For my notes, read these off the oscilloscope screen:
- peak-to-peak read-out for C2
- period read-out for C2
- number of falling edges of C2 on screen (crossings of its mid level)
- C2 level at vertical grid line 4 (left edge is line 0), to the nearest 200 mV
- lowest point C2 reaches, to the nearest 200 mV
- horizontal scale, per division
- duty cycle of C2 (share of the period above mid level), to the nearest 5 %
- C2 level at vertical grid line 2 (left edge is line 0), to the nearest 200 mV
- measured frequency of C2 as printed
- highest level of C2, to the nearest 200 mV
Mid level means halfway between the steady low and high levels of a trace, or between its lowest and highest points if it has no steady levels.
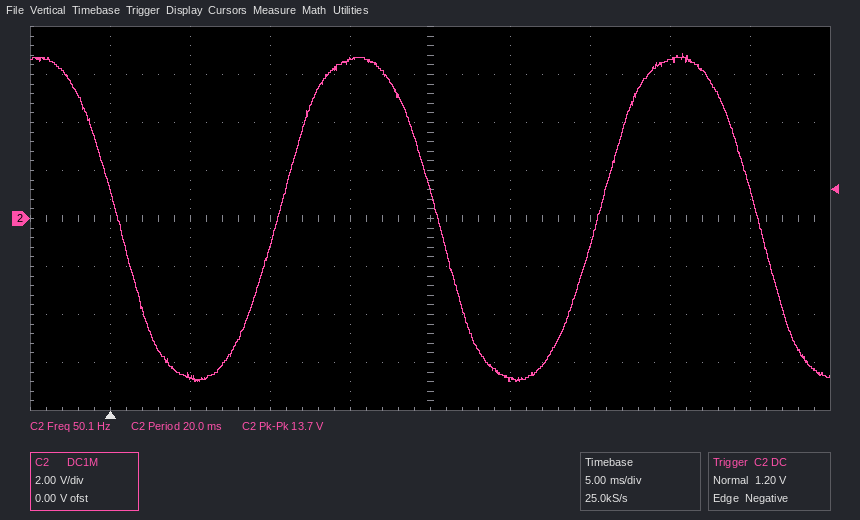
13.7 V
20.0 ms
3
6.6 V
-6.8 V
5 ms
50 %
-6.6 V
50.1 Hz
6.8 V
